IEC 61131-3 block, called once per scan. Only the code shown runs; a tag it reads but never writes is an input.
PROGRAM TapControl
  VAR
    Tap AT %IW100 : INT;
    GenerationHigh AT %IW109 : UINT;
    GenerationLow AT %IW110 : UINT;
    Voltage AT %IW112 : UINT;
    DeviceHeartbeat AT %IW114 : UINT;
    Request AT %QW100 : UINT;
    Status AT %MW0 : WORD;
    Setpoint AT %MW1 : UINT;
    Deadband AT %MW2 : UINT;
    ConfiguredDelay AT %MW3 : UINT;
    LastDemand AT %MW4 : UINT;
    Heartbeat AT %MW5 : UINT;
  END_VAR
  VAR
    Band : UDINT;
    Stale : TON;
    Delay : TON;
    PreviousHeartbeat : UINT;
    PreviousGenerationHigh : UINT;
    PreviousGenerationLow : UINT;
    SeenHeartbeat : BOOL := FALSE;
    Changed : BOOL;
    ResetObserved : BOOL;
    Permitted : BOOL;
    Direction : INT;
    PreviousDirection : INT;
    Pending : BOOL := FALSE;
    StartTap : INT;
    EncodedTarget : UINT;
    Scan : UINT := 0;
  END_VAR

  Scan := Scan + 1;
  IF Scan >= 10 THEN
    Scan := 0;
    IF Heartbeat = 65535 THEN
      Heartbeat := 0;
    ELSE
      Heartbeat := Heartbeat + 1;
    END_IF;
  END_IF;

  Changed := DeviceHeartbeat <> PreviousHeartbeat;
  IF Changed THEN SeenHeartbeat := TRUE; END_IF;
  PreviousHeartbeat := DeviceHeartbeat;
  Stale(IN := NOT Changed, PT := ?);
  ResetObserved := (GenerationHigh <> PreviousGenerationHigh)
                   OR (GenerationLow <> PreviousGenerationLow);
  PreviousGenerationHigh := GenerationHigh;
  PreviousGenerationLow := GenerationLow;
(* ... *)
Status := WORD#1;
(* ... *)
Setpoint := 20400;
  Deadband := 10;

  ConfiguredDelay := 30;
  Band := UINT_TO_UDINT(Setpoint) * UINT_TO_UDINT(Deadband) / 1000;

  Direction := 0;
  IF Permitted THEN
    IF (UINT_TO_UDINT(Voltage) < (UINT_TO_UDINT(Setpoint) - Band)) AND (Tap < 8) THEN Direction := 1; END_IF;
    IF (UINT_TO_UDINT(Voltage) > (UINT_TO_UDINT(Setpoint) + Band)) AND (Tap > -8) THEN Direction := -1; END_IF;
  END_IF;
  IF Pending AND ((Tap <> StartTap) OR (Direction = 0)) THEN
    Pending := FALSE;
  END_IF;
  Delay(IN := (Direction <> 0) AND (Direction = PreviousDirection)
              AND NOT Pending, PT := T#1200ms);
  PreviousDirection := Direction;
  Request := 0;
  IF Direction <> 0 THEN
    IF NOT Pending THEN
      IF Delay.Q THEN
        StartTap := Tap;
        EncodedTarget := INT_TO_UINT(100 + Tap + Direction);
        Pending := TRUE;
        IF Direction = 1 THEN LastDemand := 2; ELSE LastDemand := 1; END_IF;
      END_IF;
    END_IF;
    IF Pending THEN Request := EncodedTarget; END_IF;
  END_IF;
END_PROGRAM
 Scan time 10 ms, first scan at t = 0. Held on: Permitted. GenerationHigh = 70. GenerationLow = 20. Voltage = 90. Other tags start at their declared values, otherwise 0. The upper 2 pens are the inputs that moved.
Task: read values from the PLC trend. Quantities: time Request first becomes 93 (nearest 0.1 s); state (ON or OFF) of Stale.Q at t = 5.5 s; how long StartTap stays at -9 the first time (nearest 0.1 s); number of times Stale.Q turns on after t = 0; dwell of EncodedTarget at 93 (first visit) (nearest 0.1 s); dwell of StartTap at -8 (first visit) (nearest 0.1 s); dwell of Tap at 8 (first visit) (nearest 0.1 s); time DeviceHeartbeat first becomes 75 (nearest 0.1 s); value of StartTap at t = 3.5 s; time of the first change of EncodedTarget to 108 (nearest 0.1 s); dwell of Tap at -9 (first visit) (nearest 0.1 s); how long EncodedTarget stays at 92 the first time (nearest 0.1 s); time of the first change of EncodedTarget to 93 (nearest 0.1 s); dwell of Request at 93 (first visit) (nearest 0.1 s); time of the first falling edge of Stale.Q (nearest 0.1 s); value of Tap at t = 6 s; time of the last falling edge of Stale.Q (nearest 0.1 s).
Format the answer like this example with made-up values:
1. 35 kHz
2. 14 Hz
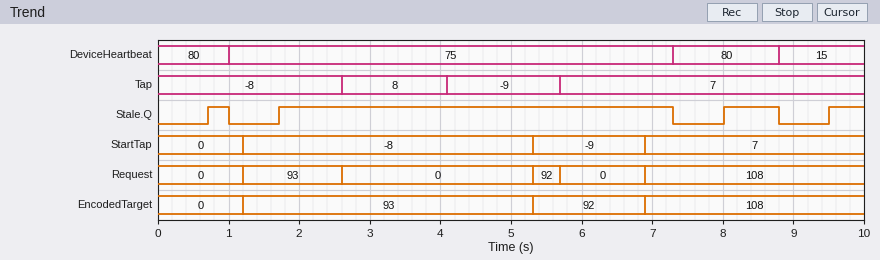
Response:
1. 1.2 s
2. ON
3. 1.6 s
4. 4
5. 4.1 s
6. 4.1 s
7. 1.5 s
8. 1.0 s
9. -8
10. 6.9 s
11. 1.6 s
12. 1.6 s
13. 1.2 s
14. 1.4 s
15. 1.0 s
16. 7
17. 8.8 s
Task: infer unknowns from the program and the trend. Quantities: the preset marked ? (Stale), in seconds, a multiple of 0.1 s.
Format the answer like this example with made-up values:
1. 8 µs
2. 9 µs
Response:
1. 0.7 s
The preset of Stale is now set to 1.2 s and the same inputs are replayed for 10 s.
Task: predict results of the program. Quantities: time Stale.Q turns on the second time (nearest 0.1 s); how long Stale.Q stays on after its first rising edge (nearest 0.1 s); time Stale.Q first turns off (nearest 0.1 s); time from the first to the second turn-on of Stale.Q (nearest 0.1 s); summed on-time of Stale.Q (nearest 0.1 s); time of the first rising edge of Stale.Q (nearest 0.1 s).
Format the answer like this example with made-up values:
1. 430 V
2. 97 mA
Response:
1. 8.5 s
2. 5.1 s
3. 7.3 s
4. 6.3 s
5. 5.4 s
6. 2.2 s
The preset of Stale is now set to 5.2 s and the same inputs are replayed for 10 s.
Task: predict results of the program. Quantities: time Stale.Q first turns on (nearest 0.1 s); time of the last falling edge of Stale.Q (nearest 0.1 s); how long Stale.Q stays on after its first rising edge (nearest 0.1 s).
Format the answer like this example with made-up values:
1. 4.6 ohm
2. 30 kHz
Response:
1. 6.2 s
2. 7.3 s
3. 1.1 s
